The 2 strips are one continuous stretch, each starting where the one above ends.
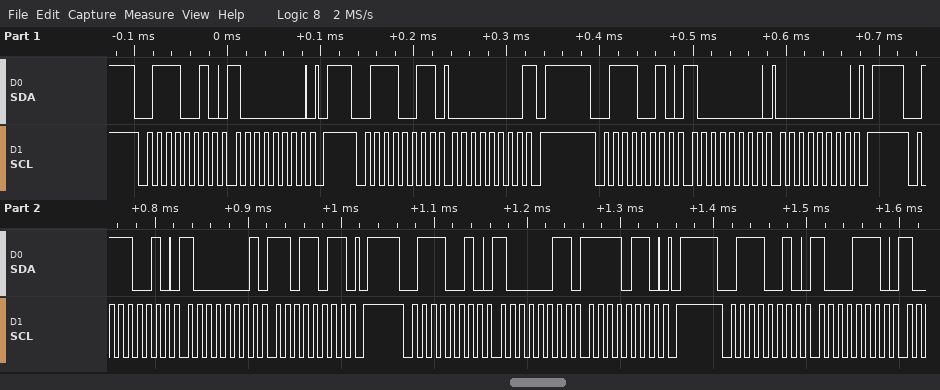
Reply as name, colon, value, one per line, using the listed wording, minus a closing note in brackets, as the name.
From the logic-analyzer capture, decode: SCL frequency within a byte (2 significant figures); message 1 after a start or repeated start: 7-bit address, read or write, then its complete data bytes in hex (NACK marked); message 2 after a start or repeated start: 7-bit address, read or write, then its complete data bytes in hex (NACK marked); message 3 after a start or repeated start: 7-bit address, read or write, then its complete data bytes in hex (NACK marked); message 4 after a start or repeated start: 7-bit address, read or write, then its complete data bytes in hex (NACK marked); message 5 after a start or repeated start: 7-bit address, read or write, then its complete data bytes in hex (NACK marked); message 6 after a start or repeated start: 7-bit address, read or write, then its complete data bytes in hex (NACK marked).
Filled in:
SCL frequency within a byte: 100 kHz
message 1 after a start or repeated start: 7-bit address, read or write, then its complete data bytes in hex: 0x39 write: 80
message 2 after a start or repeated start: 7-bit address, read or write, then its complete data bytes in hex: 0x39 read: 00 NACK
message 3 after a start or repeated start: 7-bit address, read or write, then its complete data bytes in hex: 0x39 write: 80 00
message 4 after a start or repeated start: 7-bit address, read or write, then its complete data bytes in hex: 0x39 write: 81 DB
message 5 after a start or repeated start: 7-bit address, read or write, then its complete data bytes in hex: 0x39 write: 83 F6
message 6 after a start or repeated start: 7-bit address, read or write, then its complete data bytes in hex: 0x39 write: 8E
